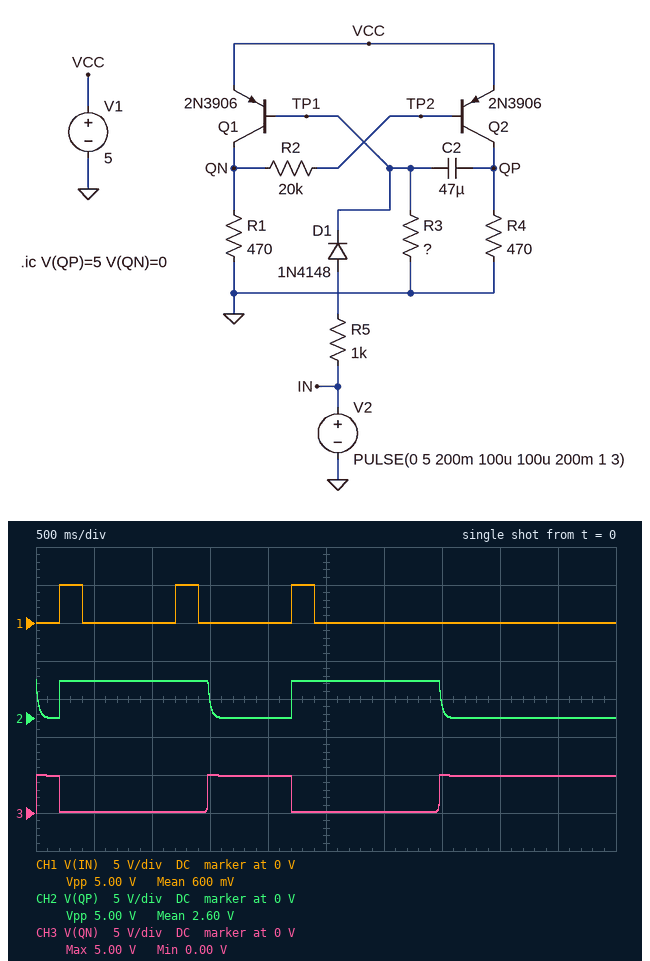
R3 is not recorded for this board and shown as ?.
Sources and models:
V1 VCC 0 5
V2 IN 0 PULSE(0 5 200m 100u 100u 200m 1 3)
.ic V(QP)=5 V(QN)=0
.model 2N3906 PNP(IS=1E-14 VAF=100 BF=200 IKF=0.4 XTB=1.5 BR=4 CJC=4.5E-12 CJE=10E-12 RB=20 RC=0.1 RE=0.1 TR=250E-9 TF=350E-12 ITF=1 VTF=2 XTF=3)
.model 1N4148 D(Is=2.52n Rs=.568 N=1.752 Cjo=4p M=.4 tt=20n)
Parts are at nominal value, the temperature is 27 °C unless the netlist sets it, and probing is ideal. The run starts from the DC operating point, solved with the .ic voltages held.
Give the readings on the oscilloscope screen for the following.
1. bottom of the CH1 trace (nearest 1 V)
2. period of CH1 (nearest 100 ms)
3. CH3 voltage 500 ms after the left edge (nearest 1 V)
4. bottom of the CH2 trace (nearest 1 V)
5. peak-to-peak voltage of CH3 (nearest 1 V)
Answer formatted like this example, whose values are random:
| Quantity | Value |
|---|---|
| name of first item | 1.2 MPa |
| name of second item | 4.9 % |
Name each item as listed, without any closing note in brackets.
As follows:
| Quantity | Value |
|---|---|
| bottom of the CH1 trace | 0 V |
| period of CH1 | 1.0 s |
| CH3 voltage 500 ms after the left edge | 0 V |
| bottom of the CH2 trace | 0 V |
| peak-to-peak voltage of CH3 | 5 V |
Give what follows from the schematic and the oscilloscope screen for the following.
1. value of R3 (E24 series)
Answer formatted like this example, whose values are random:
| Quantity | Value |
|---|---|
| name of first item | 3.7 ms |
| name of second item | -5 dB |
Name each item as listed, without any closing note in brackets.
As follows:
| Quantity | Value |
|---|---|
| value of R3 | 36 kΩ |
